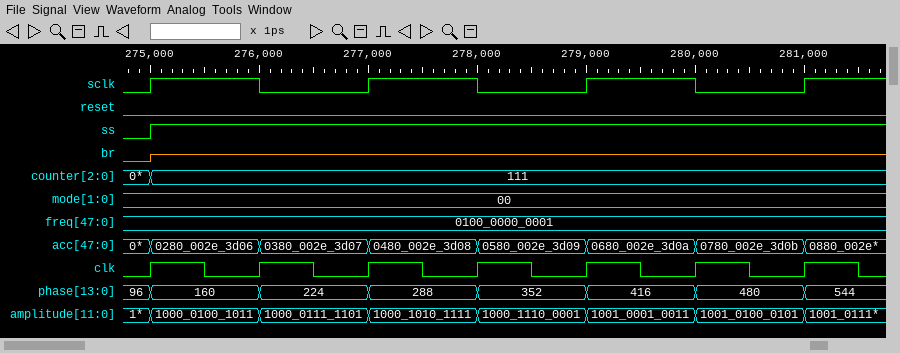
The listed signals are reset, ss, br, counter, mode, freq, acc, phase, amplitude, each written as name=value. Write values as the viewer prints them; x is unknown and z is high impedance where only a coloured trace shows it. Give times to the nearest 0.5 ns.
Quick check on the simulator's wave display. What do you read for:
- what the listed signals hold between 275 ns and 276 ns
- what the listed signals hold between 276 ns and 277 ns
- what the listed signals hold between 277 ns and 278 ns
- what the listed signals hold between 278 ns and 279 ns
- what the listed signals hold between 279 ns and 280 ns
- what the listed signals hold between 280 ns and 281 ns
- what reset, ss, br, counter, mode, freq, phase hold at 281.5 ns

reset=0, ss=1, br=z, counter=111, mode=00, freq=0100_0000_0001, acc=0280_002e_3d06, phase=160, amplitude=1000_0100_1011
reset=0, ss=1, br=z, counter=111, mode=00, freq=0100_0000_0001, acc=0380_002e_3d07, phase=224, amplitude=1000_0111_1101
reset=0, ss=1, br=z, counter=111, mode=00, freq=0100_0000_0001, acc=0480_002e_3d08, phase=288, amplitude=1000_1010_1111
reset=0, ss=1, br=z, counter=111, mode=00, freq=0100_0000_0001, acc=0580_002e_3d09, phase=352, amplitude=1000_1110_0001
reset=0, ss=1, br=z, counter=111, mode=00, freq=0100_0000_0001, acc=0680_002e_3d0a, phase=416, amplitude=1001_0001_0011
reset=0, ss=1, br=z, counter=111, mode=00, freq=0100_0000_0001, acc=0780_002e_3d0b, phase=480, amplitude=1001_0100_0101
reset=0, ss=1, br=z, counter=111, mode=00, freq=0100_0000_0001, phase=544
